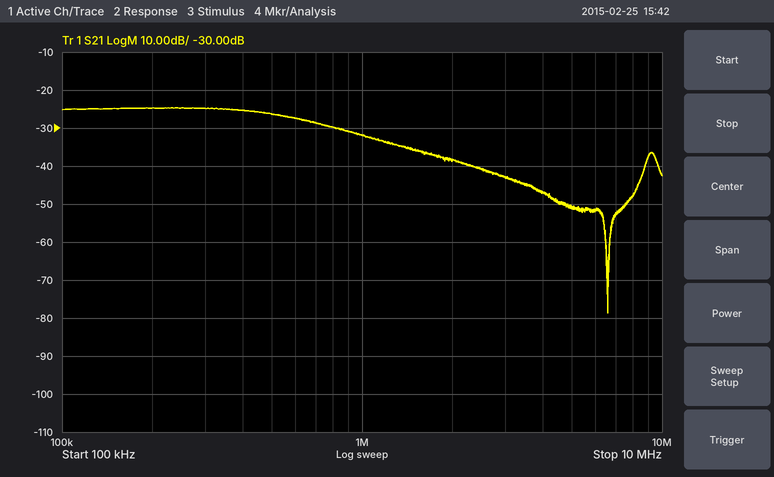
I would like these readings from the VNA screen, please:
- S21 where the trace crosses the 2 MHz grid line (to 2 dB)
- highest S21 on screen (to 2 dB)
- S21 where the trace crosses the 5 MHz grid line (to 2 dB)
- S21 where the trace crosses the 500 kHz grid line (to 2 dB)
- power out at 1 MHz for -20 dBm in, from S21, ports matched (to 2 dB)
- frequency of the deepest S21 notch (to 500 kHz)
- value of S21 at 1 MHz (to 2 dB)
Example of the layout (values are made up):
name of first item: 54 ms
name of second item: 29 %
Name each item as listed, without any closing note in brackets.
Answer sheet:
S21 where the trace crosses the 2 MHz grid line: -38 dB
highest S21 on screen: -24 dB
S21 where the trace crosses the 5 MHz grid line: -50 dB
S21 where the trace crosses the 500 kHz grid line: -26 dB
power out at 1 MHz for -20 dBm in, from S21, ports matched: -52 dBm
frequency of the deepest S21 notch: 6.5 MHz
value of S21 at 1 MHz: -32 dB
